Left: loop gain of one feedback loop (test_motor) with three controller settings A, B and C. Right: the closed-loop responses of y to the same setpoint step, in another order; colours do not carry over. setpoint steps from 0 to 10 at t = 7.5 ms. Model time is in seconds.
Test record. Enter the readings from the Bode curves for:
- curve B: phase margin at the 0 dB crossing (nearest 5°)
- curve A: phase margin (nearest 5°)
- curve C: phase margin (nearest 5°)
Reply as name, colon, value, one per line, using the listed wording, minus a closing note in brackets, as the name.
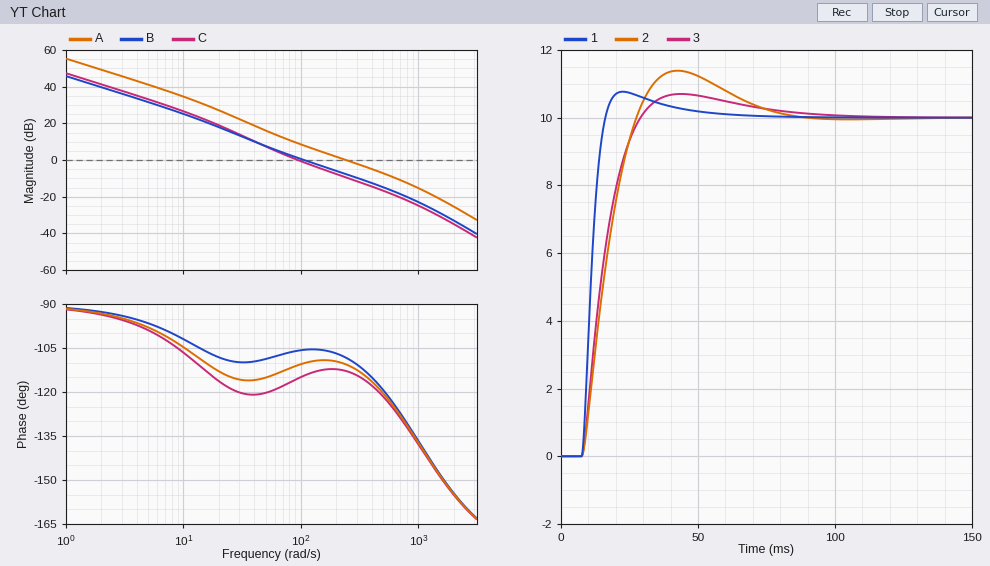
curve B: phase margin at the 0 dB crossing: 75°
curve A: phase margin: 70°
curve C: phase margin: 65°
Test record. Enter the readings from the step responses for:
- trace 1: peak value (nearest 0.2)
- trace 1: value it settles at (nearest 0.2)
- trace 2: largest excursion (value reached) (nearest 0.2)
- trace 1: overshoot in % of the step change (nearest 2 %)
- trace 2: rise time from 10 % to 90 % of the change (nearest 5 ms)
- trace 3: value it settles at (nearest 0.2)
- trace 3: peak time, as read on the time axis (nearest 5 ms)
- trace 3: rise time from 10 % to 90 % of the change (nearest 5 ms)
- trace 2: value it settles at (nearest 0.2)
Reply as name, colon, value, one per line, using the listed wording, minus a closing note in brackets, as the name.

trace 1: peak value: 10.8
trace 1: value it settles at: 10.0
trace 2: largest excursion (value reached): 11.4
trace 1: overshoot in % of the step change: 8 %
trace 2: rise time from 10 % to 90 % of the change: 15 ms
trace 3: value it settles at: 10.0
trace 3: peak time, as read on the time axis: 45 ms
trace 3: rise time from 10 % to 90 % of the change: 15 ms
trace 2: value it settles at: 10.0
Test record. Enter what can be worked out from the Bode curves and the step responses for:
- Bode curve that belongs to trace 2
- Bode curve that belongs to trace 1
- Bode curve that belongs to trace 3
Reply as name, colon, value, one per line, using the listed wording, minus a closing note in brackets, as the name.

Bode curve that belongs to trace 2: C
Bode curve that belongs to trace 1: A
Bode curve that belongs to trace 3: B
